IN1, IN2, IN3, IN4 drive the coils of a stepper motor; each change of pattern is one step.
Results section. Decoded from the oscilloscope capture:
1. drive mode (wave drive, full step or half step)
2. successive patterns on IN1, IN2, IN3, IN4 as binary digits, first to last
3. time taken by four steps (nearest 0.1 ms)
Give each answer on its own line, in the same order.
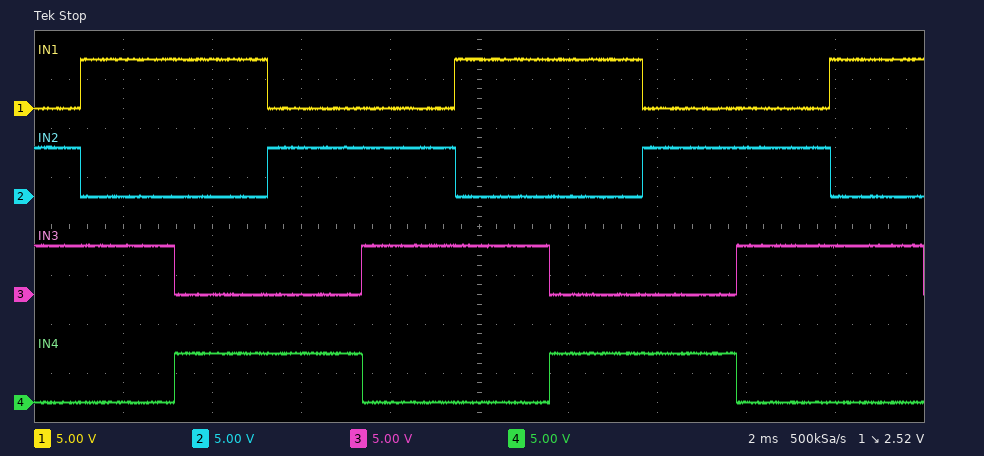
full step
0110 1010 1001 0101 0110 1010 1001 0101 0110 1010
8.4 ms
